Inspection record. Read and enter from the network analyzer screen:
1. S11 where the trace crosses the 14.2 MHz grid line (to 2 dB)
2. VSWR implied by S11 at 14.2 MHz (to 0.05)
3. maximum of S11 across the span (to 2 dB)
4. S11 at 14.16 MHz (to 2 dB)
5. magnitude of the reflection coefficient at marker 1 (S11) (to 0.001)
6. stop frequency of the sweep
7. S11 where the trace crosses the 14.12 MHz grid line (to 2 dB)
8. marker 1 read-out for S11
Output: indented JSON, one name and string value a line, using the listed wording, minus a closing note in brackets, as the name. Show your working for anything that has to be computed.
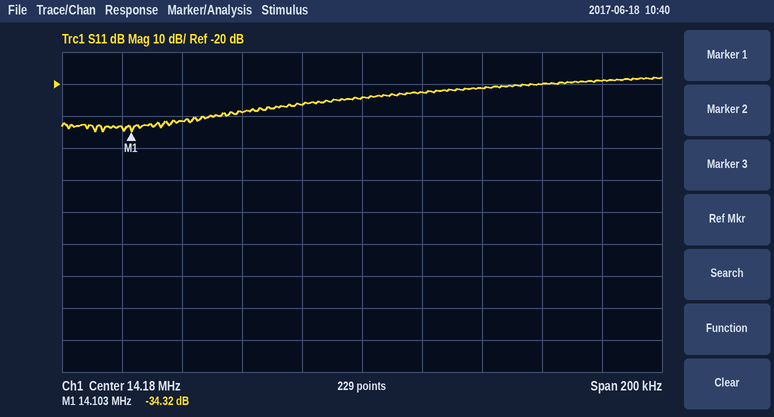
{
  "S11 where the trace crosses the 14.2 MHz grid line": "-22 dB",
  "VSWR implied by S11 at 14.2 MHz": "|Γ| = 10^(-22/20) = 0.0794; VSWR = (1 + 0.0794)/(1 − 0.0794) ≈ 1.17, so 1.15 to the nearest 0.05",
  "maximum of S11 across the span": "-18 dB",
  "S11 at 14.16 MHz": "-26 dB",
  "magnitude of the reflection coefficient at marker 1 (S11)": "10^(-34.32/20) ≈ 0.019",
  "stop frequency of the sweep": "14.28 MHz",
  "S11 where the trace crosses the 14.12 MHz grid line": "-32 dB",
  "marker 1 read-out for S11": "-34.32 dB"
}
